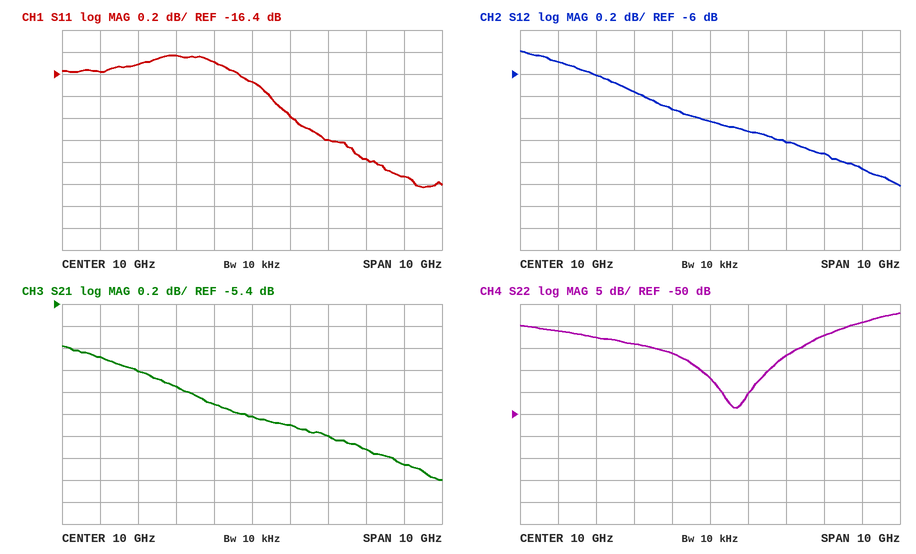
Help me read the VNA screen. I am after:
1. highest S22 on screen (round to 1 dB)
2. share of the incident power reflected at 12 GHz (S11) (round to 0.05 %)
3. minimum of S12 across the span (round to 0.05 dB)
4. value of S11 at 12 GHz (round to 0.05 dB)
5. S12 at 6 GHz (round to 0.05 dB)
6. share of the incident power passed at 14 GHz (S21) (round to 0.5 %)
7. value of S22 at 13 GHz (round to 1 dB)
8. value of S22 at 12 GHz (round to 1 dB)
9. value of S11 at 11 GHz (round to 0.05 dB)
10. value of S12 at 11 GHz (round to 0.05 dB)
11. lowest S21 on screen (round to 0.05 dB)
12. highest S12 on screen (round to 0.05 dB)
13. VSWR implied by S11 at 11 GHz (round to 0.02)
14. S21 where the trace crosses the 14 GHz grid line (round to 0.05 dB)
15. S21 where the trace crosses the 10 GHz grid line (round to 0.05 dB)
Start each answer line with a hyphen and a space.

- -27 dB
- 2.00 %
- -7.00 dB
- -17.00 dB
- -5.90 dB
- 20.5 %
- -32 dB
- -37 dB
- -16.80 dB
- -6.50 dB
- -7.00 dB
- -5.80 dB
- 1.34
- -6.85 dB
- -6.40 dB
